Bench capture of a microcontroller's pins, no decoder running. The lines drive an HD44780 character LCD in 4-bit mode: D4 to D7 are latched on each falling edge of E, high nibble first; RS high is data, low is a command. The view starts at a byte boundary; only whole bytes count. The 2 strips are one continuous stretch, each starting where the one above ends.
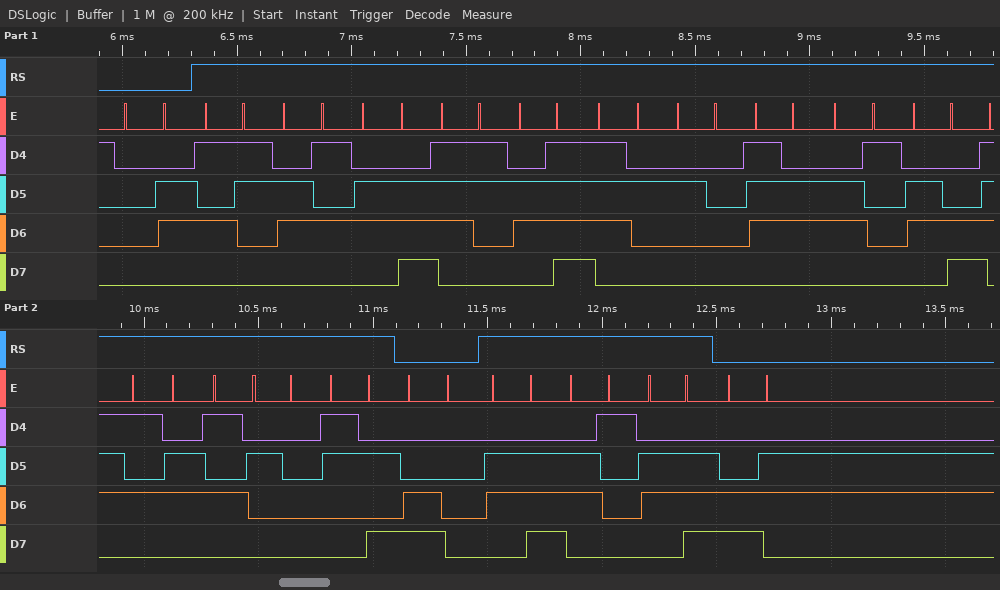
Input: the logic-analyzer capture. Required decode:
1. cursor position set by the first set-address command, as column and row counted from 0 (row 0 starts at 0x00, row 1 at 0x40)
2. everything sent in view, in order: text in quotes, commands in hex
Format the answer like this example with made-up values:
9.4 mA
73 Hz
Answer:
column 0, row 1
0x06 "Sensor value :" 0xC0 "nan" 0xC6
